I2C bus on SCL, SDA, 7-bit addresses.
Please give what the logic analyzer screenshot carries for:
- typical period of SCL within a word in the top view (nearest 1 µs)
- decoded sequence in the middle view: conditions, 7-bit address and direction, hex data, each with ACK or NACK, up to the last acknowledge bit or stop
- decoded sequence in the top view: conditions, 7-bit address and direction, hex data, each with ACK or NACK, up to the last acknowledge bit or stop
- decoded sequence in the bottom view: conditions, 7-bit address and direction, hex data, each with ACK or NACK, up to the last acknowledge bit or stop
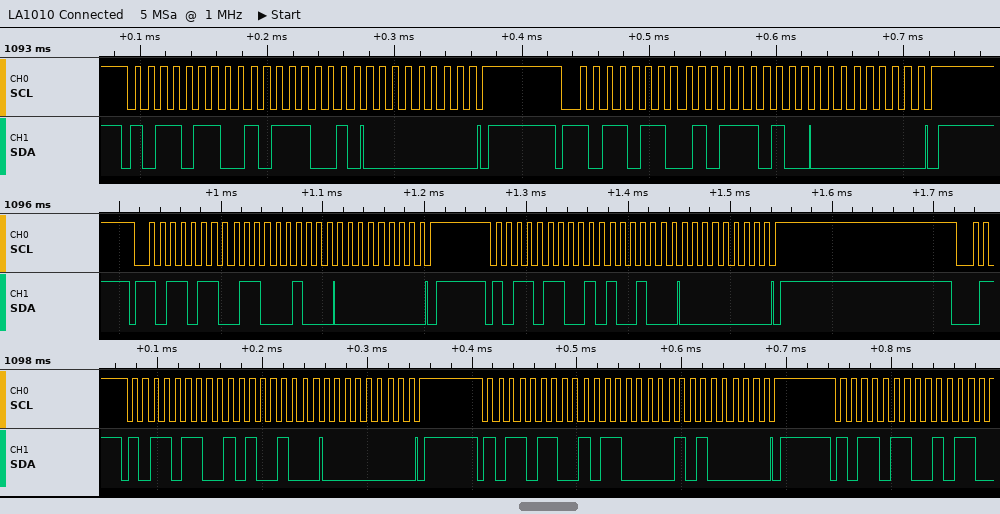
10 µs
start, address 5B write ACK, C4 ACK, 00 ACK, stop, start, address 5B write ACK, A4 ACK, 00 ACK, stop
start, address 5B write ACK, B9 ACK, 00 ACK, stop, start, address 5B write ACK, BA ACK, 00 ACK, stop
start, address 5B write ACK, A4 ACK, 00 ACK, stop, start, address 5B write ACK, B0 ACK, A0 ACK, stop, start, address 5B write ACK
